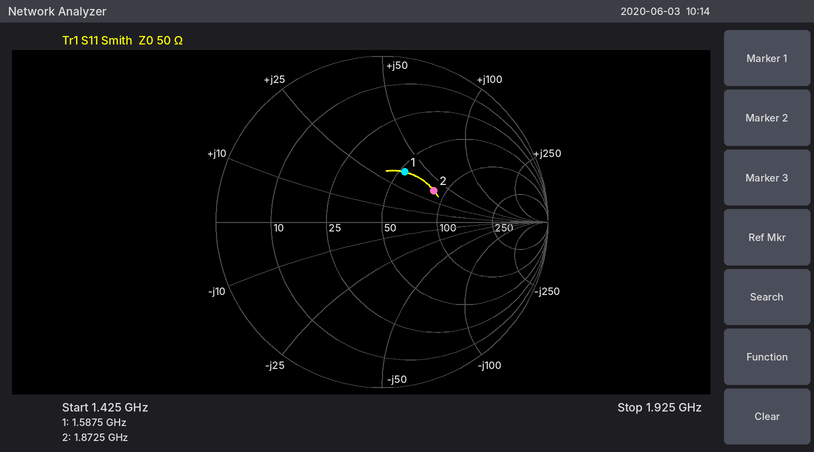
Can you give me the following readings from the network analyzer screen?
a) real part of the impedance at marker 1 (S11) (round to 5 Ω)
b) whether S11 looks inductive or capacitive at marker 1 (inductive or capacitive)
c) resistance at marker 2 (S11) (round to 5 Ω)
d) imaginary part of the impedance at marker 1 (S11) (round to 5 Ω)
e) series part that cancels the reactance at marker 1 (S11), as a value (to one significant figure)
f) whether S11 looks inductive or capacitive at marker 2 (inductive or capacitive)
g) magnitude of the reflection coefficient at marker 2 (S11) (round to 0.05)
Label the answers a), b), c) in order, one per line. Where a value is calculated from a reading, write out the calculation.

a) 55 Ω
b) inductive
c) 85 Ω
d) +35 Ω
e) C = 1/(2π × 1.5875 GHz × 35 Ω) ≈ 3 pF
f) inductive
g) 0.35
